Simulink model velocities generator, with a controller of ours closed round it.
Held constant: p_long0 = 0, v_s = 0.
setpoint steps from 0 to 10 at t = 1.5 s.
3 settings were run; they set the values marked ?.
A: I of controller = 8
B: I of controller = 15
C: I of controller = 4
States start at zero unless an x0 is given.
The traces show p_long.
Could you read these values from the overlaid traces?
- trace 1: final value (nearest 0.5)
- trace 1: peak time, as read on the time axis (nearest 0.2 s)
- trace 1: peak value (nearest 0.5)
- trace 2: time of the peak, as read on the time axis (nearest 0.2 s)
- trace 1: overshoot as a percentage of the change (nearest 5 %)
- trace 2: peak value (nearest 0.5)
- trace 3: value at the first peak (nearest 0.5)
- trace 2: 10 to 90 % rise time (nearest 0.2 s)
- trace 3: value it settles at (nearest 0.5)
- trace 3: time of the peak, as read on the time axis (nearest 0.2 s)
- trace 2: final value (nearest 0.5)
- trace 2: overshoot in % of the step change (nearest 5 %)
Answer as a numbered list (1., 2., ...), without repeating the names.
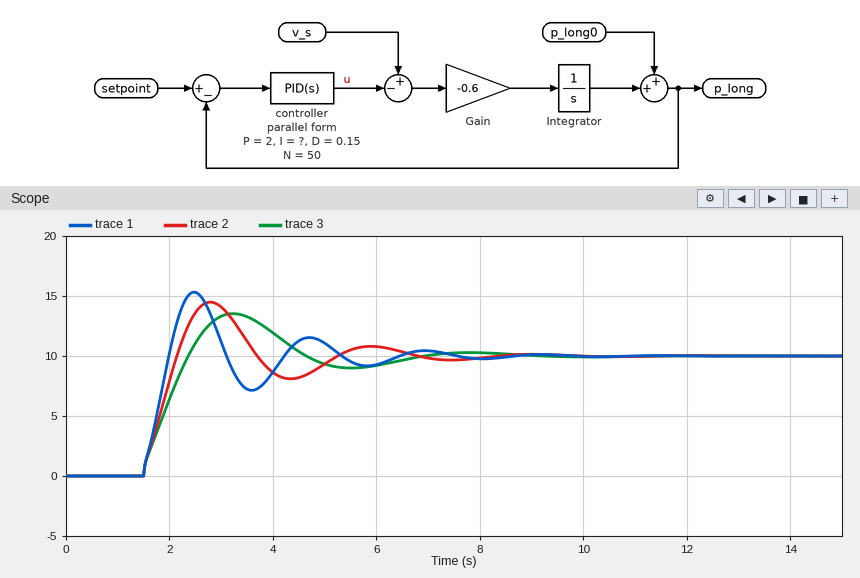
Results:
1. 10.0
2. 2.4 s
3. 15.5
4. 2.8 s
5. 55 %
6. 14.5
7. 13.5
8. 0.6 s
9. 10.0
10. 3.2 s
11. 10.0
12. 45 %
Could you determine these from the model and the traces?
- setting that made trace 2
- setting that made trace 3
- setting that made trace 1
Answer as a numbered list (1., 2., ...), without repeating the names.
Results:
1. A
2. C
3. B
